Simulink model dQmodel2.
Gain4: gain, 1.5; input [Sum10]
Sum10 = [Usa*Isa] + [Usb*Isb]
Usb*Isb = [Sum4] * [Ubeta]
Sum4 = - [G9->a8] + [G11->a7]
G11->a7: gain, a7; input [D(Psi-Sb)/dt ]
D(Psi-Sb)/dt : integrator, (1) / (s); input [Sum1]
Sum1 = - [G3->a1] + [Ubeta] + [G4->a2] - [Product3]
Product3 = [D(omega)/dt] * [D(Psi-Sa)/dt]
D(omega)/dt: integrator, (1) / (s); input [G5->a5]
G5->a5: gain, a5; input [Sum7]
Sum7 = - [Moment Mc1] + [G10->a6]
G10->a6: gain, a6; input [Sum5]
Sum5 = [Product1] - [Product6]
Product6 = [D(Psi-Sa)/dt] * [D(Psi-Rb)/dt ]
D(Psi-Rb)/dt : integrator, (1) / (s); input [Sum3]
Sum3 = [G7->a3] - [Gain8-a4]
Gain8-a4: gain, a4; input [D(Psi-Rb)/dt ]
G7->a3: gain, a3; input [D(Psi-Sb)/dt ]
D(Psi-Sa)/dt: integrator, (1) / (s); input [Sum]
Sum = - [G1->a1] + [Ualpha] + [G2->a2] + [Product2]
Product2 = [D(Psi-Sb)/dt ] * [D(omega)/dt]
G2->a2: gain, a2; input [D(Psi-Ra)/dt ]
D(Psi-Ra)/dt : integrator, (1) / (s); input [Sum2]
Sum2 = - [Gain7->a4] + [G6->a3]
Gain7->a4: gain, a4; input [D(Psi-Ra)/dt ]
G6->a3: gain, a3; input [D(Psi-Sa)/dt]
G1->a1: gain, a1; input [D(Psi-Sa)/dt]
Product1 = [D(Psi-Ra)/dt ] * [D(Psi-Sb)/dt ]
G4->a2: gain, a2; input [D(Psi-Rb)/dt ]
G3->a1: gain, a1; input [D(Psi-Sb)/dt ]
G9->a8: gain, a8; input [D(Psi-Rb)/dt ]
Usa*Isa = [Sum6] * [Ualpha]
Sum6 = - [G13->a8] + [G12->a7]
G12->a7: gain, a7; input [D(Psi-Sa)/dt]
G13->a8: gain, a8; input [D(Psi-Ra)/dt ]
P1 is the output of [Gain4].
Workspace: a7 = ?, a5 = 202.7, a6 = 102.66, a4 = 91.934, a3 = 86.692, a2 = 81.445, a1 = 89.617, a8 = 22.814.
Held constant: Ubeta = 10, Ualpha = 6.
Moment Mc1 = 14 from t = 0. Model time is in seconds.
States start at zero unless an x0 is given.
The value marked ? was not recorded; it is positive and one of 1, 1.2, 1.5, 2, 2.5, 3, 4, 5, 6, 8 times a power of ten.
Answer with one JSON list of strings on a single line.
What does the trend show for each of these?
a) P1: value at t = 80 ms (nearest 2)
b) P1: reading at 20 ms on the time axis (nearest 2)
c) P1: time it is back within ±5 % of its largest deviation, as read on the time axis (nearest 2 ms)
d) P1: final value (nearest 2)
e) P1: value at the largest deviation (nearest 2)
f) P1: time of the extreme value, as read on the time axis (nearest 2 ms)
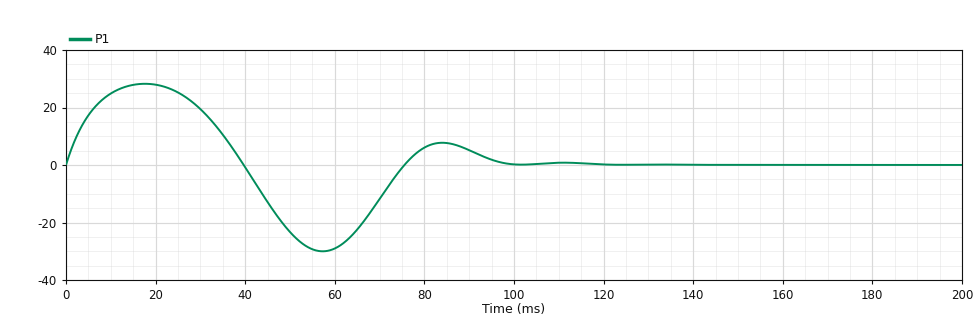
["6", "28", "96 ms", "0", "-30", "58 ms"]
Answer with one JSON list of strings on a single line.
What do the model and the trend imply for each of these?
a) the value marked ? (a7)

["25"]
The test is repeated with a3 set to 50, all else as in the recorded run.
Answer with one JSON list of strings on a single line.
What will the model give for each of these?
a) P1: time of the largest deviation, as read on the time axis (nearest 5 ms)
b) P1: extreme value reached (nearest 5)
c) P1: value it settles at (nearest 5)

["20 ms", "35", "0"]
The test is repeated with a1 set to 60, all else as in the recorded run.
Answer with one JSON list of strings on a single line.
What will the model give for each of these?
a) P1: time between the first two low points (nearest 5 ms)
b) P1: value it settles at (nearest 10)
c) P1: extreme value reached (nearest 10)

["45 ms", "0", "-70"]
